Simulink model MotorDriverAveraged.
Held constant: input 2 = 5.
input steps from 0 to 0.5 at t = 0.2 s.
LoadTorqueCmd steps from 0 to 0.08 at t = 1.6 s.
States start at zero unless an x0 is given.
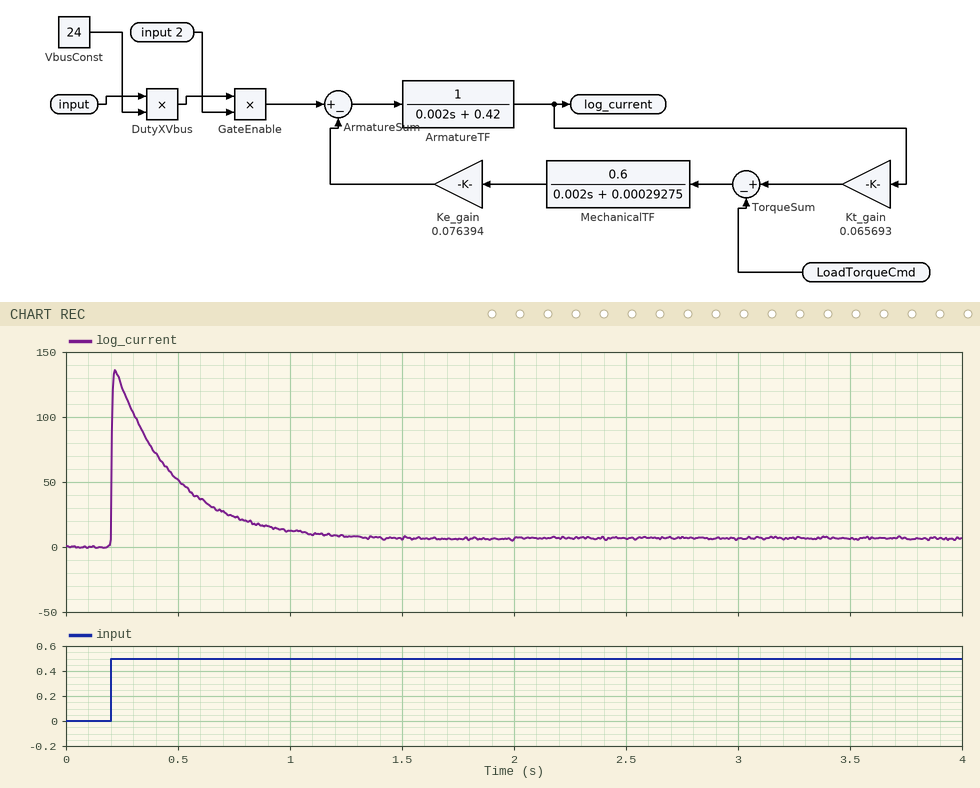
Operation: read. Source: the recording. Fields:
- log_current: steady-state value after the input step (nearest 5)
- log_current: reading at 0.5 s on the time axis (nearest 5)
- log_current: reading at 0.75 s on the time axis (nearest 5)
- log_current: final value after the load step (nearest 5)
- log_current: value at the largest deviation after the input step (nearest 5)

5
50
25
5
135
